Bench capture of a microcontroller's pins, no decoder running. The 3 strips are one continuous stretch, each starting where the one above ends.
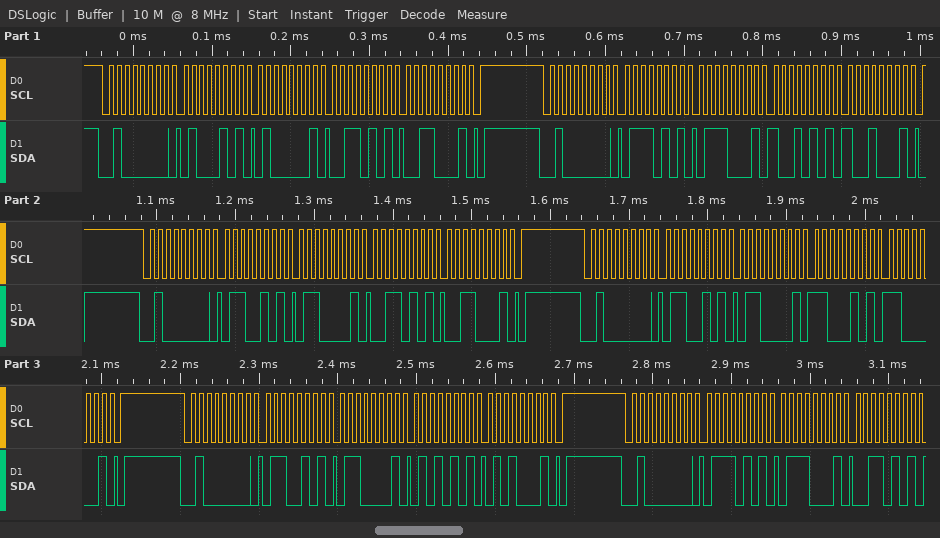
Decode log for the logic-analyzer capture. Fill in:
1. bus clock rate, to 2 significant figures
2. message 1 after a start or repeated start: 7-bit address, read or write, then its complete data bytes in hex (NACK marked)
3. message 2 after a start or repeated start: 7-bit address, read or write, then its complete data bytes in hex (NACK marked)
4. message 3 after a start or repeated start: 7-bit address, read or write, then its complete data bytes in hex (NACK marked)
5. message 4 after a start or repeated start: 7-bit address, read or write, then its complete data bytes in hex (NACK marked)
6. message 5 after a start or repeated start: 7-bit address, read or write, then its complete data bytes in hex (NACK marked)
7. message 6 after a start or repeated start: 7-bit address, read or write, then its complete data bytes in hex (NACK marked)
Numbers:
100 kHz
0x20 write: 45 41 35 31
0x20 write: 75 71 95 91
0x20 write: 65 61 35 31
0x20 write: 65 61 C5 C1
0x20 write: 65 61 55 51
0x20 write: 75 71 35
